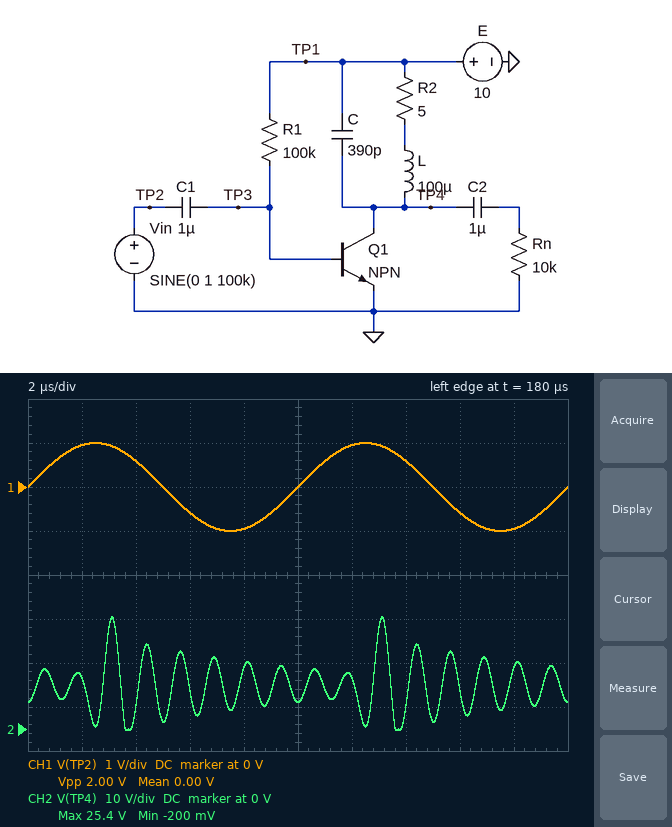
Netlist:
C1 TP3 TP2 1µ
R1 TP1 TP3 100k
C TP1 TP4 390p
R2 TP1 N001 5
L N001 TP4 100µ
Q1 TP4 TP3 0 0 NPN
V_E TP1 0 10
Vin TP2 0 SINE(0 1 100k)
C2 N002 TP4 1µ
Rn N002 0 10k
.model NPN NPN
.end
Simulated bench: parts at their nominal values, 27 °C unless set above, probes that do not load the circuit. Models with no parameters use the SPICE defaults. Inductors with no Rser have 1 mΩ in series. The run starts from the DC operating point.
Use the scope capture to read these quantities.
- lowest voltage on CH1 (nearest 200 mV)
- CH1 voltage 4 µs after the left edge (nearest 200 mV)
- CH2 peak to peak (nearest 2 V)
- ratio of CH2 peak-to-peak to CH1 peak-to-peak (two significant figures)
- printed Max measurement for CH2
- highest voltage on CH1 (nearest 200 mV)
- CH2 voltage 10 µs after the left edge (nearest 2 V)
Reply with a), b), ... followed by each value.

a) -1.0 V
b) 600 mV
c) 26 V
d) 13
e) 25.4 V
f) 1.0 V
g) 6 V
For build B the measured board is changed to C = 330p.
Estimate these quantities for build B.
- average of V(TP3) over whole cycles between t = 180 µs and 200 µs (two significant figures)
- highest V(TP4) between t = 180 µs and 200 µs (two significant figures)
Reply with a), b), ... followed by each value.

a) -140 mV
b) 26 V
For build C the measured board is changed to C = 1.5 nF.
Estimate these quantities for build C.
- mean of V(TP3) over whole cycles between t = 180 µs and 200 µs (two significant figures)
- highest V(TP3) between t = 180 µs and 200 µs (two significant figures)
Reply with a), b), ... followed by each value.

a) -170 mV
b) 830 mV
